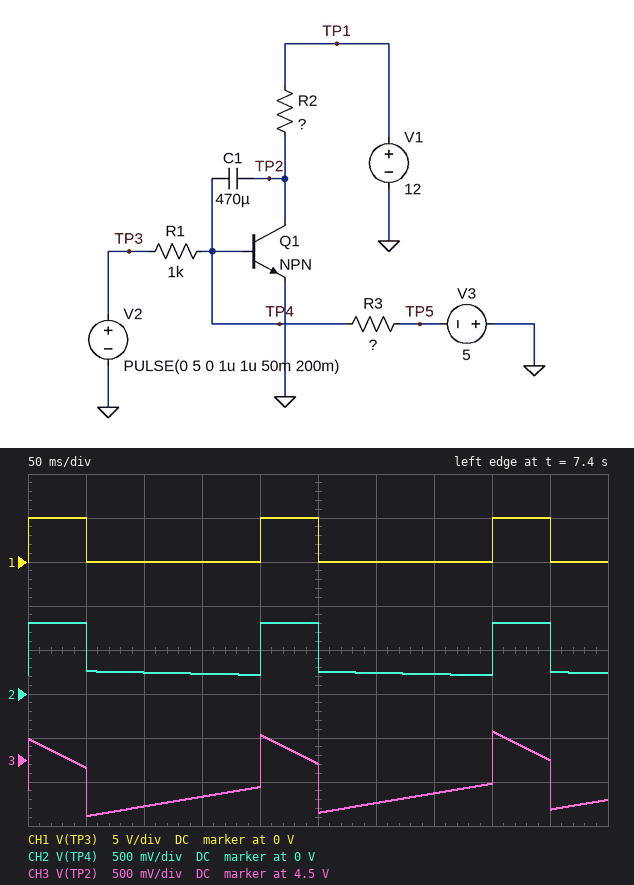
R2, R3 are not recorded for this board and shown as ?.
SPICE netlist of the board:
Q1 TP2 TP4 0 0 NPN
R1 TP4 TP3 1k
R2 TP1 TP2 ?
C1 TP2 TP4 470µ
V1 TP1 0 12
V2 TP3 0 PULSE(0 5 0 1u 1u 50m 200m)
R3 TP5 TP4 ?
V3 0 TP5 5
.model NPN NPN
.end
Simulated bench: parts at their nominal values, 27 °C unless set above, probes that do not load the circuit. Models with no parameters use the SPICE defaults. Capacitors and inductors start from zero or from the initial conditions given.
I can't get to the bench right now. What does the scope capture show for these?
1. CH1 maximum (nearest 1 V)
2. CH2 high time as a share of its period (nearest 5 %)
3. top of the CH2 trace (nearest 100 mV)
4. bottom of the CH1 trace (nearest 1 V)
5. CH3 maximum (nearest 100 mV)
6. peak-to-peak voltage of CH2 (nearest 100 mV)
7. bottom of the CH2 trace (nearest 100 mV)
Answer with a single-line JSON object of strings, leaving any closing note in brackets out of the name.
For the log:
{"CH1 maximum": "5 V", "CH2 high time as a share of its period": "25 %", "top of the CH2 trace": "800 mV", "bottom of the CH1 trace": "0 V", "CH3 maximum": "4.8 V", "peak-to-peak voltage of CH2": "600 mV", "bottom of the CH2 trace": "200 mV"}
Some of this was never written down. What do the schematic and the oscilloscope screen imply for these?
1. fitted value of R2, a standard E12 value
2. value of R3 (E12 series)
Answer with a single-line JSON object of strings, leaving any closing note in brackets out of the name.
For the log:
{"fitted value of R2, a standard E12 value": "6.8 kΩ", "value of R3": "5.6 kΩ"}
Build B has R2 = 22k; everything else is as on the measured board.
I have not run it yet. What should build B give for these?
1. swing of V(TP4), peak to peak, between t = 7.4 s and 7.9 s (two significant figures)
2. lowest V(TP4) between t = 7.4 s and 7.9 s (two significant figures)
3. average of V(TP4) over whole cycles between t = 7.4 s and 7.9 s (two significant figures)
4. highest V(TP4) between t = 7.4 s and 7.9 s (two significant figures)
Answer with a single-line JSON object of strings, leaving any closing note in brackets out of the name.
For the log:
{"swing of V(TP4), peak to peak, between t = 7.4 s and 7.9 s": "1.1 V", "lowest V(TP4) between t = 7.4 s and 7.9 s": "-260 mV", "average of V(TP4) over whole cycles between t = 7.4 s and 7.9 s": "64 mV", "highest V(TP4) between t = 7.4 s and 7.9 s": "820 mV"}
